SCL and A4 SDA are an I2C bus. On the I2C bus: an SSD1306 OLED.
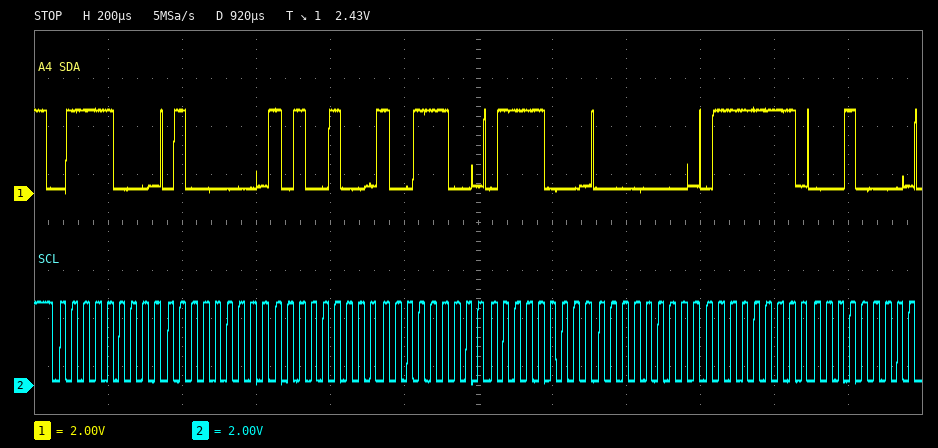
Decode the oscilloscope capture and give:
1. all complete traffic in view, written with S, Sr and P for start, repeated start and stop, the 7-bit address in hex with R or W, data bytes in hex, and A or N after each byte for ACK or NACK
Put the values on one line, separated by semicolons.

S 3CW A 40 A A4 A 9C A 78 A 00 A 7F A 10 A
